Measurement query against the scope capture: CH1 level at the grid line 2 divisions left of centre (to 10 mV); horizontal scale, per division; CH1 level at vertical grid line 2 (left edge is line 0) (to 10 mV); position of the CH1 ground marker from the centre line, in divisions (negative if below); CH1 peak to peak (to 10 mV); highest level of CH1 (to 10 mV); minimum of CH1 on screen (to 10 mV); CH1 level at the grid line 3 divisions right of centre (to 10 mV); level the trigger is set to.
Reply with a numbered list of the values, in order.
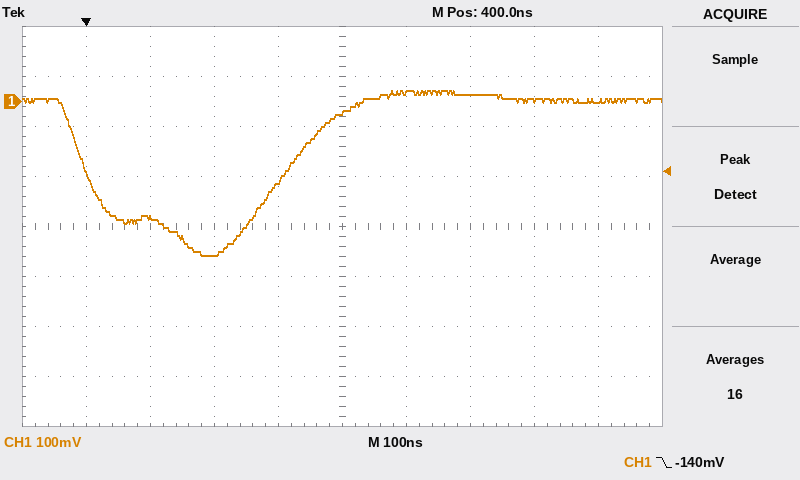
1. -310 mV
2. 100 ns
3. -230 mV
4. +2.5 div
5. 330 mV
6. 20 mV
7. -310 mV
8. 0 mV
9. -140 mV
